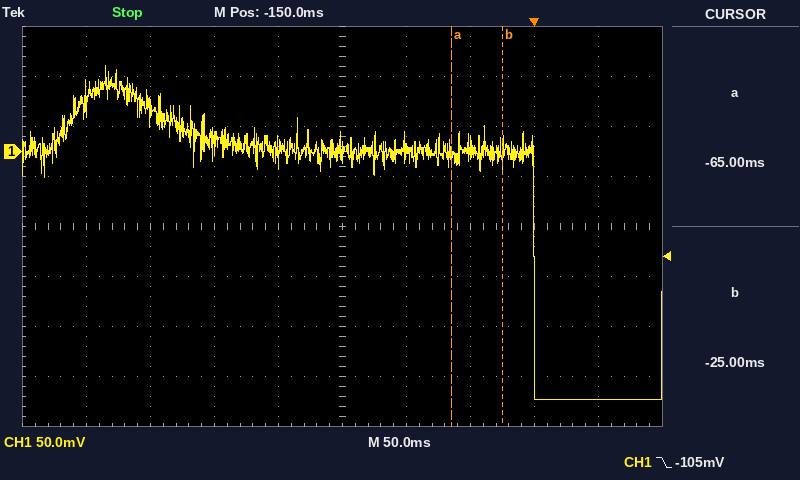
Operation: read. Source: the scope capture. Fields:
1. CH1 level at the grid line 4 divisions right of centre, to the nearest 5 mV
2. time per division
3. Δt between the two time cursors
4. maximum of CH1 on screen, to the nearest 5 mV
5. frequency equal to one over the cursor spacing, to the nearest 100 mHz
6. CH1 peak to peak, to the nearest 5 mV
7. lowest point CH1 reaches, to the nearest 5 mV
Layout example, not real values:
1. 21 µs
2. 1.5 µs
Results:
1. -250 mV
2. 50 ms
3. 40 ms
4. 85 mV
5. 25.0 Hz
6. 335 mV
7. -250 mV
